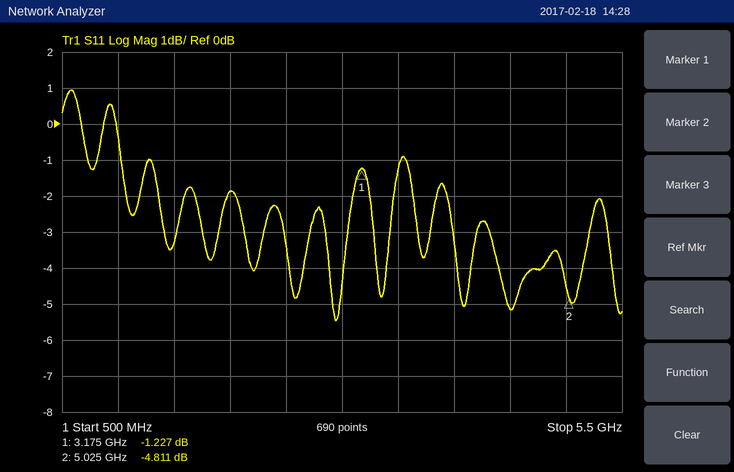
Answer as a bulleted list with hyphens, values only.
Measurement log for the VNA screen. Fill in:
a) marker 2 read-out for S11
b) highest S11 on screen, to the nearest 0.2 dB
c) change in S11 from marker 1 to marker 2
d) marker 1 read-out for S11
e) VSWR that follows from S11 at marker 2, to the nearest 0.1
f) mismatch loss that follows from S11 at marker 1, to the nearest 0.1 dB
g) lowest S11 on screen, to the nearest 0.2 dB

- -4.811 dB
- 1.0 dB
- -3.584 dB
- -1.227 dB
- 3.7
- 6.1 dB
- -5.4 dB
